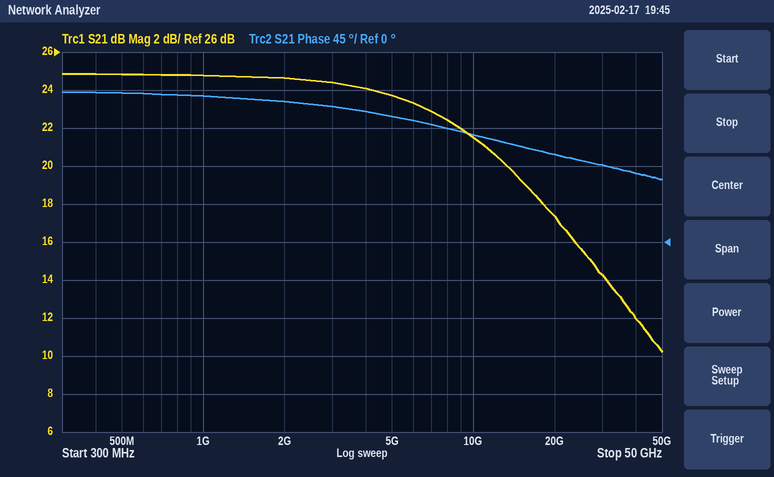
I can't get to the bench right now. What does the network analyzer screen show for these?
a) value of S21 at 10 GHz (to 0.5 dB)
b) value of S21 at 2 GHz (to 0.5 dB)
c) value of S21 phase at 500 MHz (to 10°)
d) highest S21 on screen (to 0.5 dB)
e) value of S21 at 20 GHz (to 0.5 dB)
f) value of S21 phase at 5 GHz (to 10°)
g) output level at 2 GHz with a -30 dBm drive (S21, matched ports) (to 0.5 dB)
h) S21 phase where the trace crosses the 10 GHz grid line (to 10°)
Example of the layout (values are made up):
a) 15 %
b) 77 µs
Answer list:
a) 21.5 dB
b) 24.5 dB
c) 180°
d) 25.0 dB
e) 17.5 dB
f) 150°
g) -5.5 dBm
h) 130°
